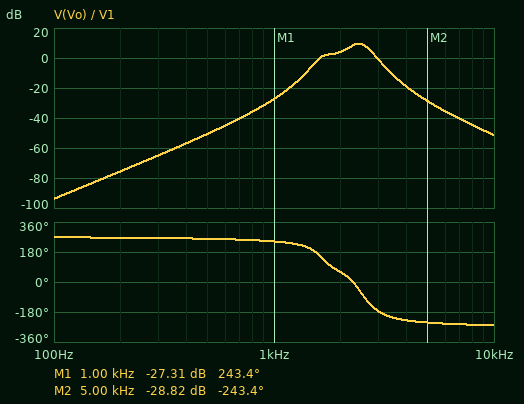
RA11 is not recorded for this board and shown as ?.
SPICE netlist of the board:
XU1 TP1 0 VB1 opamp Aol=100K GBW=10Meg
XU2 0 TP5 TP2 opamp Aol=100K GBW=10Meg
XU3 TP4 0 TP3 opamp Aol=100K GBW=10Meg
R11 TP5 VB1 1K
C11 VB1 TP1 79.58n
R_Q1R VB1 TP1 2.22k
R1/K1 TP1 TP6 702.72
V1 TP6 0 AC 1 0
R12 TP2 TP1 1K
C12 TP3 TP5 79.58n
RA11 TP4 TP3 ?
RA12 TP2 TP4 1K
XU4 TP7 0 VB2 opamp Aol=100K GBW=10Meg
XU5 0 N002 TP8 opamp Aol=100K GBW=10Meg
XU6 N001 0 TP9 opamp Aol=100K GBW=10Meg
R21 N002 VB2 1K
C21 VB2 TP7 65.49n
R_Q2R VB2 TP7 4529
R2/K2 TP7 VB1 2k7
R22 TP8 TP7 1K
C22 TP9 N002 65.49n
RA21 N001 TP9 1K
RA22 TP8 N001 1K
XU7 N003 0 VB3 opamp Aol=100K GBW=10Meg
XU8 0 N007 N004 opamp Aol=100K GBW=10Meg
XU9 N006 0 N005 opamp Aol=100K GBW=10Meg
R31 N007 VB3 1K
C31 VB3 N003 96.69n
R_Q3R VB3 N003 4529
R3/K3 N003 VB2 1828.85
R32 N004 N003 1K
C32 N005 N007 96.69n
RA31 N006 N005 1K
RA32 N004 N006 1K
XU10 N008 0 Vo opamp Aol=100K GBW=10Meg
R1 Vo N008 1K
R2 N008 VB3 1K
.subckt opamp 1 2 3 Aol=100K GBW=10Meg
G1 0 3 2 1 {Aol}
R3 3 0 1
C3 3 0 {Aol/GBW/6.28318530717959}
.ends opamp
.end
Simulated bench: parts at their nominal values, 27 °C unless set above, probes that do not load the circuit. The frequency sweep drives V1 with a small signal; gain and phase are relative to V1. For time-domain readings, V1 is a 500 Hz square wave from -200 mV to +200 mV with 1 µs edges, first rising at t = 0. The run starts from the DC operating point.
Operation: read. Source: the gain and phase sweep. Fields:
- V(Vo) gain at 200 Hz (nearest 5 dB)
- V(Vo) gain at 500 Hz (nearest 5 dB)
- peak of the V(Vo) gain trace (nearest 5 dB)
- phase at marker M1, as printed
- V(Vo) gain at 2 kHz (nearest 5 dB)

-75 dB
-50 dB
10 dB
243.4 deg
5 dB
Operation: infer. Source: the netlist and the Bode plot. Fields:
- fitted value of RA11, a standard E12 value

560 Ω
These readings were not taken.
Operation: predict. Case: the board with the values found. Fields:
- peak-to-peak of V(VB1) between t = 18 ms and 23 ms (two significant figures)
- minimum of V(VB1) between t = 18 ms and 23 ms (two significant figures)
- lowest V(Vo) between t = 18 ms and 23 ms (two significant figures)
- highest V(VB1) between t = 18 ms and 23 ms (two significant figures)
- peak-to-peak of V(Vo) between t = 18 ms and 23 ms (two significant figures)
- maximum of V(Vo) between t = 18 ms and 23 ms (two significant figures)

700 mV
-350 mV
-190 mV
350 mV
380 mV
190 mV
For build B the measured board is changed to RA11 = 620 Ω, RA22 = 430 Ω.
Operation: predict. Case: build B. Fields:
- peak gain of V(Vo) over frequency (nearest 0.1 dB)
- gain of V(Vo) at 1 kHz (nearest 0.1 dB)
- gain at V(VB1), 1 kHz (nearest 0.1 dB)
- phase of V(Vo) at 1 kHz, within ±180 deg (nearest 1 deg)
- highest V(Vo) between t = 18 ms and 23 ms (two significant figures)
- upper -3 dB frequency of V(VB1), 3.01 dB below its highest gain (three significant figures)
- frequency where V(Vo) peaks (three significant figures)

13.6 dB
-16.7 dB
-5.8 dB
-131 deg
280 mV
3.03 kHz
1.66 kHz
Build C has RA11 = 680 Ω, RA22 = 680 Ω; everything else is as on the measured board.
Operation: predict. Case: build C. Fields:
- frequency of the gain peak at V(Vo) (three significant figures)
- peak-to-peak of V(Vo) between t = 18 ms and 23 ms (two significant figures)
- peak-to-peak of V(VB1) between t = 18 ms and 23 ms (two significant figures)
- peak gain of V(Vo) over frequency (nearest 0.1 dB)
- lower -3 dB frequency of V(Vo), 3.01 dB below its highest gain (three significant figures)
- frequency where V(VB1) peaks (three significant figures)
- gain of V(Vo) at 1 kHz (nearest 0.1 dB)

1.95 kHz
400 mV
750 mV
13.1 dB
1.65 kHz
2.42 kHz
-21.2 dB
